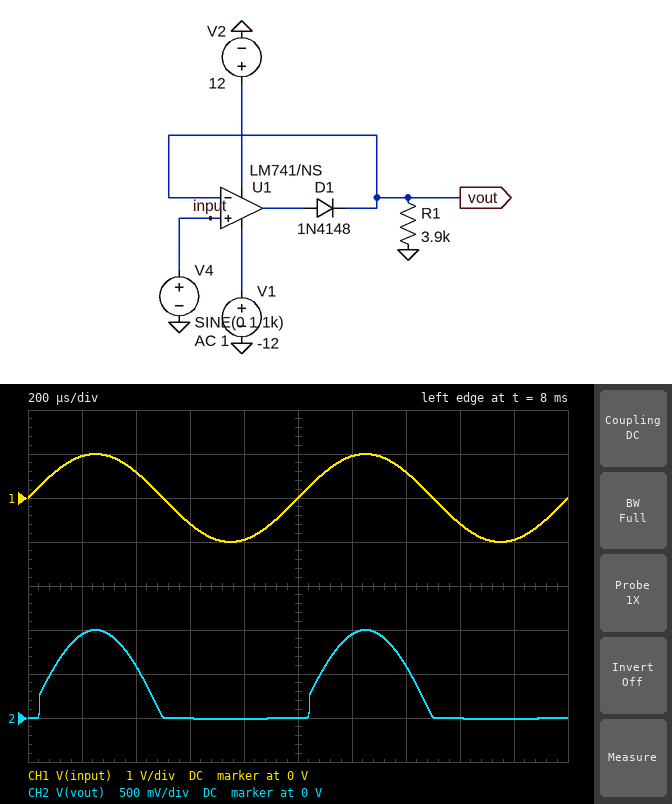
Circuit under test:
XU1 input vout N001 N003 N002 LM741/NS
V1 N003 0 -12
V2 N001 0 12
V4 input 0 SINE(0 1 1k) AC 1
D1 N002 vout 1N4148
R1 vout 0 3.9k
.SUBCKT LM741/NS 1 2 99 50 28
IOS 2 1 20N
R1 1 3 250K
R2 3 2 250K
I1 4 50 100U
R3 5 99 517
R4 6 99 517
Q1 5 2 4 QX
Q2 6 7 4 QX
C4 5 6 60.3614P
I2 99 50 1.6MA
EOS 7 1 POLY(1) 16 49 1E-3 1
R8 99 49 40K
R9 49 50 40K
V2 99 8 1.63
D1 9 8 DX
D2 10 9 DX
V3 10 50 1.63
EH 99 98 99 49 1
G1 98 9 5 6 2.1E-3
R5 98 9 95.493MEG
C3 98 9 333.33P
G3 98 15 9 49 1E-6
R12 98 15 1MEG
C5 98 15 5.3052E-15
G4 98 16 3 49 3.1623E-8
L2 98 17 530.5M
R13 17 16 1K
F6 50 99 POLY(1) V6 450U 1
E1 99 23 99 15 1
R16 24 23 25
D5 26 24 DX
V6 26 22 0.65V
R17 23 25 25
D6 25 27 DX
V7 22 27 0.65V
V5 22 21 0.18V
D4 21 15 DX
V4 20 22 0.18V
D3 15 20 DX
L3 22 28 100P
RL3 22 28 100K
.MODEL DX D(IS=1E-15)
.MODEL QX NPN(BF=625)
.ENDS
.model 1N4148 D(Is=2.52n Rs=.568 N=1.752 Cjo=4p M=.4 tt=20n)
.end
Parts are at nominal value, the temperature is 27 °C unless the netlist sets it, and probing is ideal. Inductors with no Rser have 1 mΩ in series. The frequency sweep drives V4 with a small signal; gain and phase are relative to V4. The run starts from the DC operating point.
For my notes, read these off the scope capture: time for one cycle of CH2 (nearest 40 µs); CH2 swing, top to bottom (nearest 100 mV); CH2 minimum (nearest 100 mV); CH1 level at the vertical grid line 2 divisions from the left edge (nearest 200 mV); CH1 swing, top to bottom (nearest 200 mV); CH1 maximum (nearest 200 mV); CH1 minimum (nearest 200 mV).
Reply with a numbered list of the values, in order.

1. 1.00 ms
2. 1.0 V
3. 0 V
4. 600 mV
5. 2.0 V
6. 1.0 V
7. -1.0 V
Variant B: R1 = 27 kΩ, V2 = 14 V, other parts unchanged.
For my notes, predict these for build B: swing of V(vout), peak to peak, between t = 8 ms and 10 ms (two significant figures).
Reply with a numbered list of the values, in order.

1. 1.1 V
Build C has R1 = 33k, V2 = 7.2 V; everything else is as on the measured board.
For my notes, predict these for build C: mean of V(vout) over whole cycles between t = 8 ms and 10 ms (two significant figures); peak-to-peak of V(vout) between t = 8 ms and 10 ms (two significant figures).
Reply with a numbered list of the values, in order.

1. 290 mV
2. 1.1 V
